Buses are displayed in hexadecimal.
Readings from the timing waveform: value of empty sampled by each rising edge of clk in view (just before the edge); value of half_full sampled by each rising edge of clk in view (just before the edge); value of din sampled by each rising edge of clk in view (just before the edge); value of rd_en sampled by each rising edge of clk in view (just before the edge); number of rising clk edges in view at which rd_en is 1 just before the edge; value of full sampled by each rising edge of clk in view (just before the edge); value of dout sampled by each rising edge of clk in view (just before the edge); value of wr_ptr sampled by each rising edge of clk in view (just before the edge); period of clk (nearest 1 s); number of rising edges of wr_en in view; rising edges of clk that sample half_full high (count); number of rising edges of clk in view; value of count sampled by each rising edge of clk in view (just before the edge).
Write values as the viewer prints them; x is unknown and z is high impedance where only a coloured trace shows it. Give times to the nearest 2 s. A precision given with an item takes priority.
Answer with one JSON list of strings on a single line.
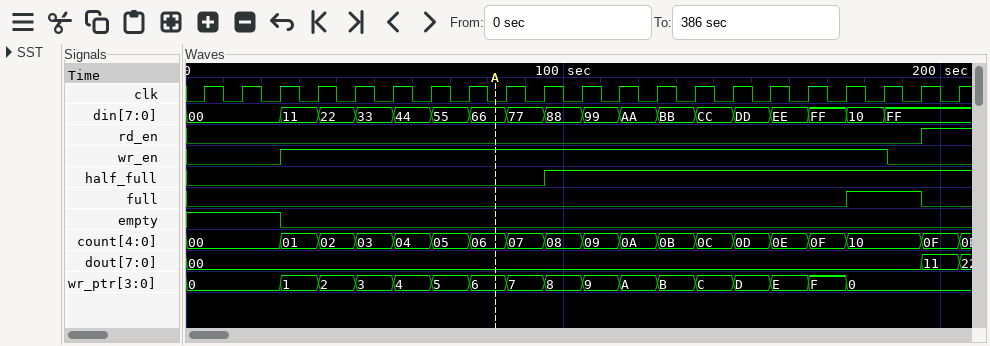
["1 1 1 0 0 0 0 0 0 0 0 0 0 0 0 0 0 0 0 0 0", "0 0 0 0 0 0 0 0 0 0 1 1 1 1 1 1 1 1 1 1 1", "00, 00, 00, 11, 22, 33, 44, 55, 66, 77, 88, 99, AA, BB, CC, DD, EE, FF, 10, FF, FF", "0 0 0 0 0 0 0 0 0 0 0 0 0 0 0 0 0 0 0 0 1", "1", "0 0 0 0 0 0 0 0 0 0 0 0 0 0 0 0 0 0 1 1 0", "00, 00, 00, 00, 00, 00, 00, 00, 00, 00, 00, 00, 00, 00, 00, 00, 00, 00, 00, 00, 11", "0, 0, 0, 1, 2, 3, 4, 5, 6, 7, 8, 9, A, B, C, D, E, F, 0, 0, 0", "10 s", "1", "11", "21", "00, 00, 00, 01, 02, 03, 04, 05, 06, 07, 08, 09, 0A, 0B, 0C, 0D, 0E, 0F, 10, 10, 0F"]
